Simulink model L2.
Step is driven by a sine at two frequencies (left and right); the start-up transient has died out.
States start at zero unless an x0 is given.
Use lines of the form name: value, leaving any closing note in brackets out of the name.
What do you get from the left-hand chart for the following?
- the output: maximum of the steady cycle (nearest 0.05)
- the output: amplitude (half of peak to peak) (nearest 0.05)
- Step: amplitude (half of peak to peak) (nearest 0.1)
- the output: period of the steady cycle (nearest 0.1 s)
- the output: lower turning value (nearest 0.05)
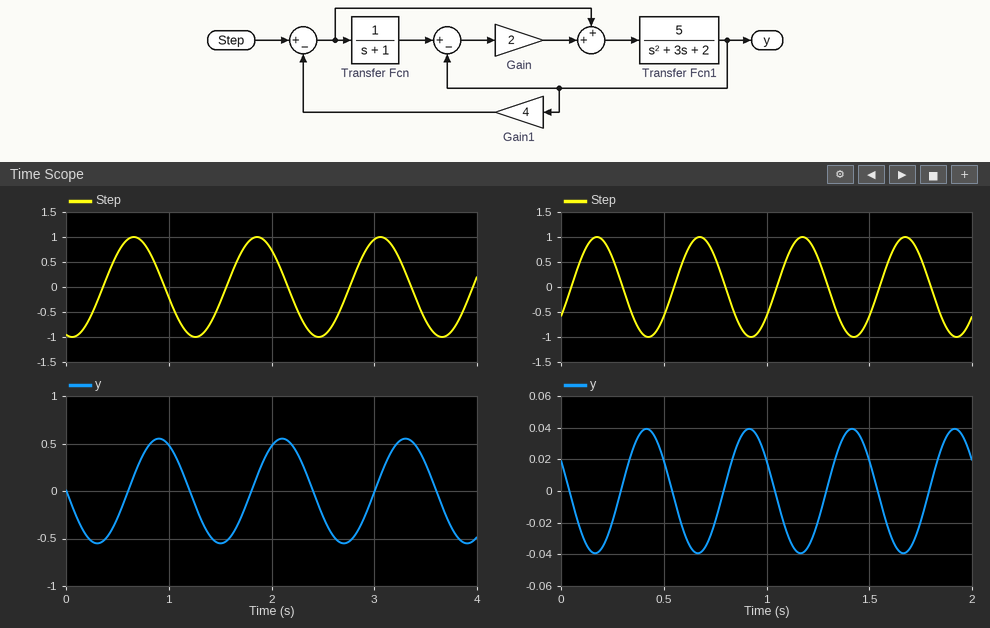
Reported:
the output: maximum of the steady cycle: 0.55
the output: amplitude (half of peak to peak): 0.55
Step: amplitude (half of peak to peak): 1.0
the output: period of the steady cycle: 1.2 s
the output: lower turning value: -0.55
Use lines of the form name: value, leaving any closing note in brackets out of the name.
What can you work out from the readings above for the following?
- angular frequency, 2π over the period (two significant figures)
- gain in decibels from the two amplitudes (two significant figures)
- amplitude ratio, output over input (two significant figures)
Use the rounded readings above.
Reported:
angular frequency, 2π over the period: 5.2 rad/s
gain in decibels from the two amplitudes: -5.2 dB
amplitude ratio, output over input: 0.55
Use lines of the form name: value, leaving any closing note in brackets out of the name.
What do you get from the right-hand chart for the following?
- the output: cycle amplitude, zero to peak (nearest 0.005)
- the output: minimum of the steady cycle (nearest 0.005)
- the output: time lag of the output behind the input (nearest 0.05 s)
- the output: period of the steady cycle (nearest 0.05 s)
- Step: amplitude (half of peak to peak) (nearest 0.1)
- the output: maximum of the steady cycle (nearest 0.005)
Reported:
the output: cycle amplitude, zero to peak: 0.040
the output: minimum of the steady cycle: -0.040
the output: time lag of the output behind the input: 0.25 s
the output: period of the steady cycle: 0.50 s
Step: amplitude (half of peak to peak): 1.0
the output: maximum of the steady cycle: 0.040
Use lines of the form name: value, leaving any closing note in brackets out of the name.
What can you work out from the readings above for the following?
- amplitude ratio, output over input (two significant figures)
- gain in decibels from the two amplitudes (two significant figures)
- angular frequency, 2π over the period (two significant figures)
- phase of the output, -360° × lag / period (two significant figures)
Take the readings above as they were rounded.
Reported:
amplitude ratio, output over input: 0.040
gain in decibels from the two amplitudes: -28 dB
angular frequency, 2π over the period: 13 rad/s
phase of the output, -360° × lag / period: -180°
